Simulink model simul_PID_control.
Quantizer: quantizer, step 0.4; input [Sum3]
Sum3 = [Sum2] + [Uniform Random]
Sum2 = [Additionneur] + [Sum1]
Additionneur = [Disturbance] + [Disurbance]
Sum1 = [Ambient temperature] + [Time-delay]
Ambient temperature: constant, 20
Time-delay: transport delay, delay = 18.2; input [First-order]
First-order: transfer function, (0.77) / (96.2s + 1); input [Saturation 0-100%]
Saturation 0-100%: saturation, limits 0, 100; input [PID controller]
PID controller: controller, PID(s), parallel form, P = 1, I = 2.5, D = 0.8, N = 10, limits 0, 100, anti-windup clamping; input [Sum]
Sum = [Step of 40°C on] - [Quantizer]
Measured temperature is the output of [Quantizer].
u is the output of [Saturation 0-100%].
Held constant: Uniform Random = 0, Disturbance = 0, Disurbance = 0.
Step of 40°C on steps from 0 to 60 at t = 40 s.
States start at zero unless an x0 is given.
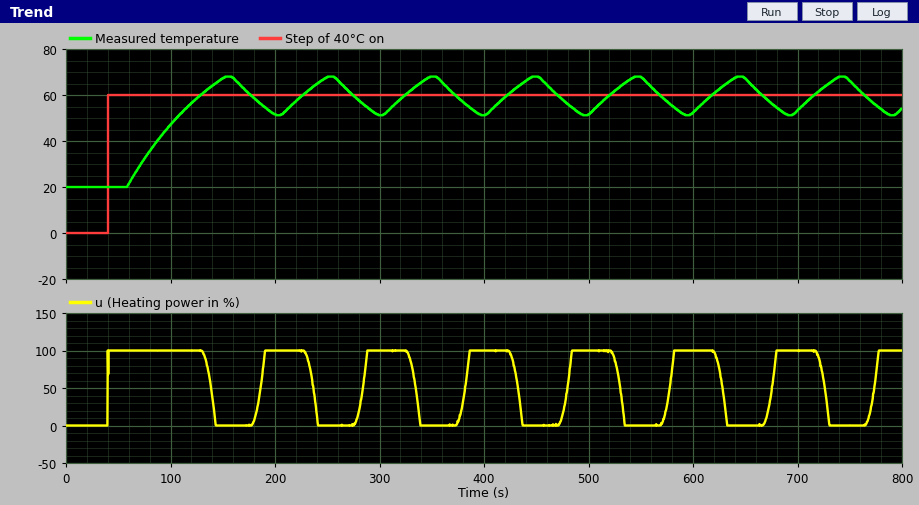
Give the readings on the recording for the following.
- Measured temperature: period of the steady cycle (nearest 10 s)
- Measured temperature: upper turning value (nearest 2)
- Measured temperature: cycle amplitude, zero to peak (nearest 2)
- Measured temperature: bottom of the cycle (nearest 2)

100 s
68
8
52
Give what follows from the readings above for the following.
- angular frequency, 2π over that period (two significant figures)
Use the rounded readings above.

0.063 rad/s
